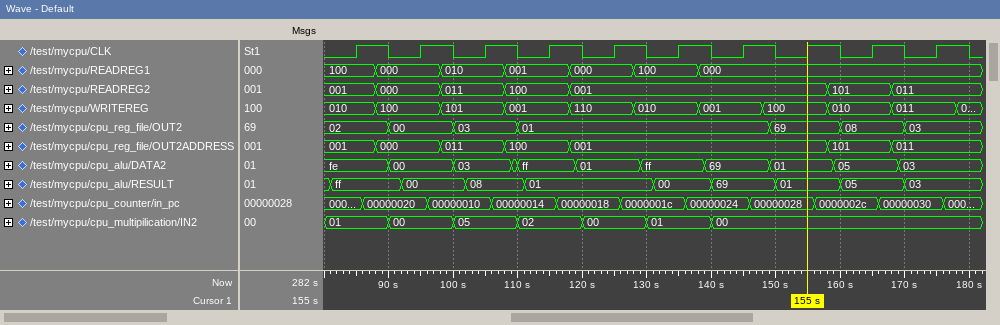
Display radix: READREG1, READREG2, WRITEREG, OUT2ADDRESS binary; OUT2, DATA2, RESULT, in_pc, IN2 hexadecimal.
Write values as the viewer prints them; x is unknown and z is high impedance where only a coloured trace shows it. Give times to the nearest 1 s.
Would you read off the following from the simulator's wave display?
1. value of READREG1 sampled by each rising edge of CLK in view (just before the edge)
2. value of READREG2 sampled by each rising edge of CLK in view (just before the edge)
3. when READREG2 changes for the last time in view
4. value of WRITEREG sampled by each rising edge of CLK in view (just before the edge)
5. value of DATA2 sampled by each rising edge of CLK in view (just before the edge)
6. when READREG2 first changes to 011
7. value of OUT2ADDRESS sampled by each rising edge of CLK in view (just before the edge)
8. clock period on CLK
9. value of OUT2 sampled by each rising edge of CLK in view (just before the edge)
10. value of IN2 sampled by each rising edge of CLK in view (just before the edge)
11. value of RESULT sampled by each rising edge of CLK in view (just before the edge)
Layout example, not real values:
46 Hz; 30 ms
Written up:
100, 000, 010, 001, 000, 100, 000, 000, 000, 000; 001, 000, 011, 100, 001, 001, 001, 001, 101, 011; 168 s; 010, 100, 101, 001, 110, 010, 001, 100, 010, 011; fe, 00, 03, ff, 01, ff, 69, 01, 05, 03; 98 s; 001, 000, 011, 100, 001, 001, 001, 001, 101, 011; 10 s; 02, 00, 03, 01, 01, 01, 01, 69, 08, 03; 01, 00, 05, 02, 00, 01, 00, 00, 00, 00; ff, 00, 08, 01, 01, 00, 69, 01, 05, 03
